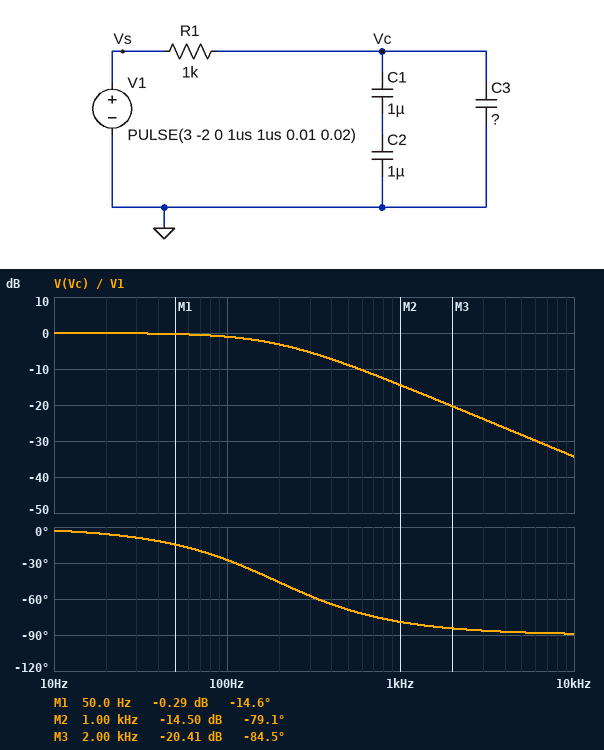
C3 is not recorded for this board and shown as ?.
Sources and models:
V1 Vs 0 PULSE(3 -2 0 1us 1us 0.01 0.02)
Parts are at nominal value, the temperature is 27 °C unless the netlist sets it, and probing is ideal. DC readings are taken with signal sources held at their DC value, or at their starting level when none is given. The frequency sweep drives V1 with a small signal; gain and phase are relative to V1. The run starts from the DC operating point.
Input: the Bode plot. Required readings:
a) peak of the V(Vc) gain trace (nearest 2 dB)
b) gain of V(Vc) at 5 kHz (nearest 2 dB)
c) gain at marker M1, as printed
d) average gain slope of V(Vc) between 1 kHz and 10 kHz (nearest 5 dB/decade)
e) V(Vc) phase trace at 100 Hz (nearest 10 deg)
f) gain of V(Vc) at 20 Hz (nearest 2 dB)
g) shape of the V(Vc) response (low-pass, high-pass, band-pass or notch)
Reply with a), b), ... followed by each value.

a) 0 dB
b) -28 dB
c) -0.29 dB
d) -20 dB/decade
e) -30 deg
f) 0 dB
g) low-pass
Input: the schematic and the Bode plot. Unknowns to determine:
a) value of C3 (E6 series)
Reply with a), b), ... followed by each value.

a) 330 nF
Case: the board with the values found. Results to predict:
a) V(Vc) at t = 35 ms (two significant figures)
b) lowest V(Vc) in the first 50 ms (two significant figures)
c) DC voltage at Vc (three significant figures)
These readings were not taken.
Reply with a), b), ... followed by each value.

a) 3.0 V
b) -2.0 V
c) 3.00 V
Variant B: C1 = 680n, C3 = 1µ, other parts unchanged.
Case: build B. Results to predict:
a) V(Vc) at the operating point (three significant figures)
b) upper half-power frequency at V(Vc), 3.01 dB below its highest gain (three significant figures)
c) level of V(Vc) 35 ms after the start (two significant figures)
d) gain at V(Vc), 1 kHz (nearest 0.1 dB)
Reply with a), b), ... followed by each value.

a) 3.00 V
b) 113 Hz
c) 2.9 V
d) -19.0 dB
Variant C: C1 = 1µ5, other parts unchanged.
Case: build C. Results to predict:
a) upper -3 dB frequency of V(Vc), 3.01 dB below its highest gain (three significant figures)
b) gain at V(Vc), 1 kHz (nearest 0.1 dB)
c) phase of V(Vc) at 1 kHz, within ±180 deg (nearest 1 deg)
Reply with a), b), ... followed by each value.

a) 171 Hz
b) -15.5 dB
c) -80 deg
